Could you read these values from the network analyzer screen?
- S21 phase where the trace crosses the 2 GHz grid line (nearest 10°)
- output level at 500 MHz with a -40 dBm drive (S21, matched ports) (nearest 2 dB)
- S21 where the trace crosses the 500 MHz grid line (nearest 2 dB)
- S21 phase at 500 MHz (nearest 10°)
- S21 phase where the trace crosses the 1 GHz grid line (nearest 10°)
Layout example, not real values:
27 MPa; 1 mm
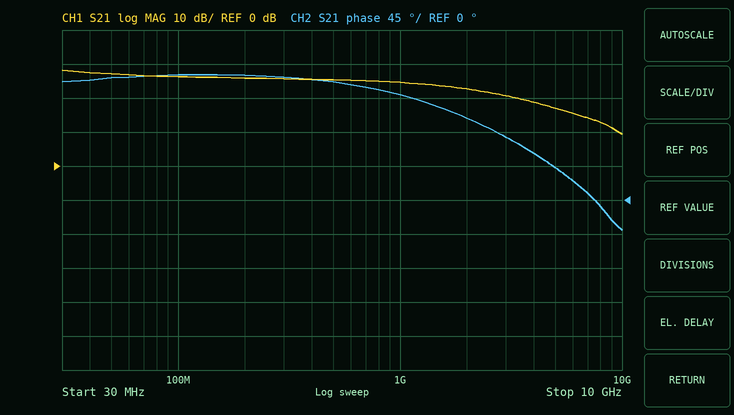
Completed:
110°; -14 dBm; 26 dB; 160°; 140°
